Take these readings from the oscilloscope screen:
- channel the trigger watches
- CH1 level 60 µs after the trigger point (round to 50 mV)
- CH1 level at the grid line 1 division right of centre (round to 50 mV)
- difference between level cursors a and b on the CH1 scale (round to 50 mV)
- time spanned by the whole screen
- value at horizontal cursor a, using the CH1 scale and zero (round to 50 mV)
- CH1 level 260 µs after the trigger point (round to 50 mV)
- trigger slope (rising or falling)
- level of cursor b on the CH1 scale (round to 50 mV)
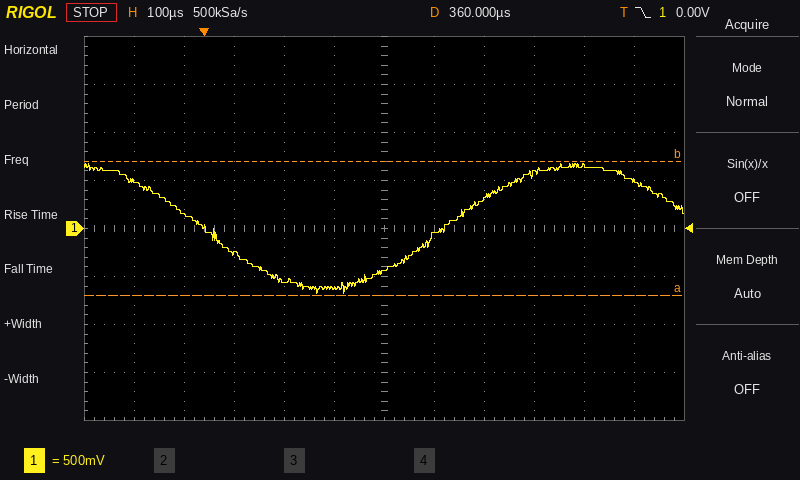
CH1
-250 mV
-50 mV
1.40 V
1.2 ms
-700 mV
-600 mV
falling
700 mV
